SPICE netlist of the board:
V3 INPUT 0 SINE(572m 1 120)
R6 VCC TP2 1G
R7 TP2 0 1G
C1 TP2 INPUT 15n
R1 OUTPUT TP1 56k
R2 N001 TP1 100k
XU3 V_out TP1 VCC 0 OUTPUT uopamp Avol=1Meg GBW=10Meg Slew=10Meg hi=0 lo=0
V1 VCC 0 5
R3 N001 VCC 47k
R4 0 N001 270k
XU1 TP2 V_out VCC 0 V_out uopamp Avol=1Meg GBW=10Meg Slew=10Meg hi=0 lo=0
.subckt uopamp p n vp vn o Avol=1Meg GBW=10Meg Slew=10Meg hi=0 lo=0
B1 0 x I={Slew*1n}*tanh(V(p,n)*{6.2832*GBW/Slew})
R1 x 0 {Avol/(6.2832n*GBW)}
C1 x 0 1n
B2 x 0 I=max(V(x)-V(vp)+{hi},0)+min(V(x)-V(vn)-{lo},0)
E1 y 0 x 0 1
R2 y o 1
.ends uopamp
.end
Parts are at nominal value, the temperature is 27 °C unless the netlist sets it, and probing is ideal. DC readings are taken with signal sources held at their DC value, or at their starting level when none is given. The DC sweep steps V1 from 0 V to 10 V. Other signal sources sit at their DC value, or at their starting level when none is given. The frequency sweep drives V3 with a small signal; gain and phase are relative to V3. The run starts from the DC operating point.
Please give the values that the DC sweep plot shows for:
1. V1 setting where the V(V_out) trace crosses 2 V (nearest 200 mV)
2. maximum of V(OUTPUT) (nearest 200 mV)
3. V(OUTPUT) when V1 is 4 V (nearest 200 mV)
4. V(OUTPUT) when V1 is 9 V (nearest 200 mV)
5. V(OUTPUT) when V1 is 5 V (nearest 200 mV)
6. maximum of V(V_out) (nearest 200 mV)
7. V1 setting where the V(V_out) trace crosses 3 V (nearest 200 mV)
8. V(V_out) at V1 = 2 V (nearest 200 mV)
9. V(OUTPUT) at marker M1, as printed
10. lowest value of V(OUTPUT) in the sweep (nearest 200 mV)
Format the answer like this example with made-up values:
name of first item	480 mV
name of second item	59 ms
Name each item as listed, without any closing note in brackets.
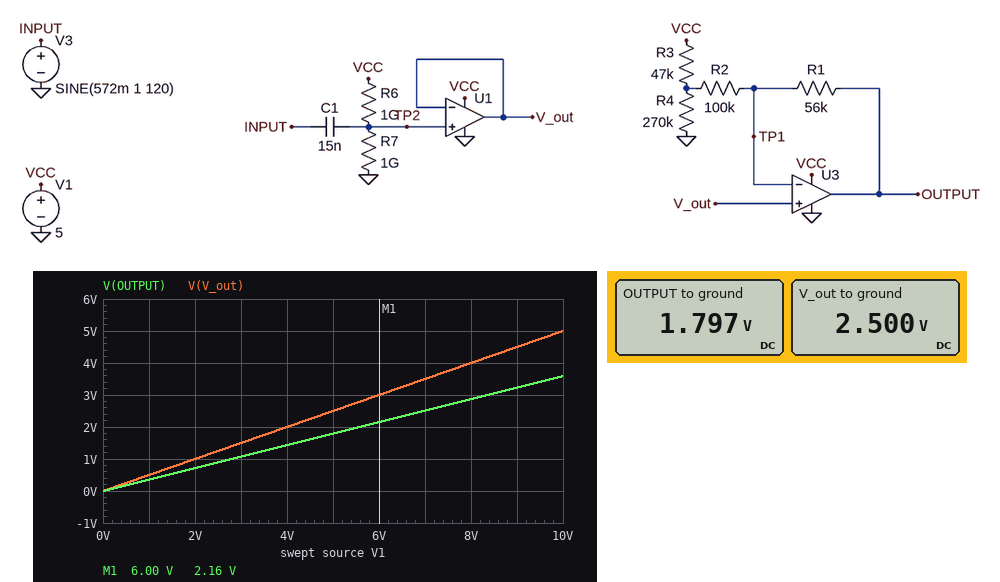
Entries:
V1 setting where the V(V_out) trace crosses 2 V	4.0 V
maximum of V(OUTPUT)	3.6 V
V(OUTPUT) when V1 is 4 V	1.4 V
V(OUTPUT) when V1 is 9 V	3.2 V
V(OUTPUT) when V1 is 5 V	1.8 V
maximum of V(V_out)	5.0 V
V1 setting where the V(V_out) trace crosses 3 V	6.0 V
V(V_out) at V1 = 2 V	1.0 V
V(OUTPUT) at marker M1, as printed	2.16 V
lowest value of V(OUTPUT) in the sweep	0 V
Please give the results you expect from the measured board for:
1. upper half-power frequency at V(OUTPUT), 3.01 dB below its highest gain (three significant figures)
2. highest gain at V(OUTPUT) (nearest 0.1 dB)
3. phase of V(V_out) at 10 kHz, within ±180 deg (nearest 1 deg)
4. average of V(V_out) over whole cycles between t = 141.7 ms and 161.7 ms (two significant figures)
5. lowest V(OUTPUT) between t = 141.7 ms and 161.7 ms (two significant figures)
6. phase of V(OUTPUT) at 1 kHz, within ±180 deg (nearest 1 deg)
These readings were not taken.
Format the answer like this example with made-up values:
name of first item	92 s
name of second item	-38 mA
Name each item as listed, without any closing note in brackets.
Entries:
upper half-power frequency at V(OUTPUT), 3.01 dB below its highest gain	5.33 MHz
highest gain at V(OUTPUT)	2.9 dB
phase of V(V_out) at 10 kHz, within ±180 deg	0 deg
average of V(V_out) over whole cycles between t = 141.7 ms and 161.7 ms	2.5 V
lowest V(OUTPUT) between t = 141.7 ms and 161.7 ms	400 mV
phase of V(OUTPUT) at 1 kHz, within ±180 deg	0 deg
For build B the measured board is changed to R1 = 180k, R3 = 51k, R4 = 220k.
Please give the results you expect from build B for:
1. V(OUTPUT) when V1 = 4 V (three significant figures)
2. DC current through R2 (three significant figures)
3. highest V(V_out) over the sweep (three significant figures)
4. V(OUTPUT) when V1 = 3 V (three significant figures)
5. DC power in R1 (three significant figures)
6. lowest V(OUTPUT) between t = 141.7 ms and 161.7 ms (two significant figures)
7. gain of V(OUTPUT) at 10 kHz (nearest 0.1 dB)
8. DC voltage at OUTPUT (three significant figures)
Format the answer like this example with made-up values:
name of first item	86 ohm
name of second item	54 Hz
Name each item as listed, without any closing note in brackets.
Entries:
V(OUTPUT) when V1 = 4 V	412 mV
DC current through R2	11.0 µA
highest V(V_out) over the sweep	5.00 V
V(OUTPUT) when V1 = 3 V	309 mV
DC power in R1	21.9 µW
lowest V(OUTPUT) between t = 141.7 ms and 161.7 ms	-10 mV
gain of V(OUTPUT) at 10 kHz	7.1 dB
DC voltage at OUTPUT	515 mV
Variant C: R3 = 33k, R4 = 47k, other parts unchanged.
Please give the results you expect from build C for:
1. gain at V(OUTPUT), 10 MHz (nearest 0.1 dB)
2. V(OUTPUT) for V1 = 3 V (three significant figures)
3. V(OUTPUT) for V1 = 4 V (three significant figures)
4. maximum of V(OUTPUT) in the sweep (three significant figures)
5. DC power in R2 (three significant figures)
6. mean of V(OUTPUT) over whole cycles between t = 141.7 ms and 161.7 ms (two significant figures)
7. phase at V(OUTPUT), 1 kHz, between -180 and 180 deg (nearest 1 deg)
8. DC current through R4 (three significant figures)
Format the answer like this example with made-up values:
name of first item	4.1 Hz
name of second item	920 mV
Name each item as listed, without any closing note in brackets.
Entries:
gain at V(OUTPUT), 10 MHz	-4.7 dB
V(OUTPUT) for V1 = 3 V	1.38 V
V(OUTPUT) for V1 = 4 V	1.84 V
maximum of V(OUTPUT) in the sweep	4.59 V
DC power in R2	1.34 µW
mean of V(OUTPUT) over whole cycles between t = 141.7 ms and 161.7 ms	2.3 V
phase at V(OUTPUT), 1 kHz, between -180 and 180 deg	0 deg
DC current through R4	61.0 µA
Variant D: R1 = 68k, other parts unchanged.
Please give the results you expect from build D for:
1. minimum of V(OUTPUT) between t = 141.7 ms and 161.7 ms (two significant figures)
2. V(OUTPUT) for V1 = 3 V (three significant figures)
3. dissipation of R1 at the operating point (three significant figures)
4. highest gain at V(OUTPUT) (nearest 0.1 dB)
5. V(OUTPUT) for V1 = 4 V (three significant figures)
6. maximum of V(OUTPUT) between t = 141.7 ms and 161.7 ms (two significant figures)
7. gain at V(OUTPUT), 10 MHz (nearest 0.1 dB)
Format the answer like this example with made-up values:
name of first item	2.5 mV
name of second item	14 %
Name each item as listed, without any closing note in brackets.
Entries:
minimum of V(OUTPUT) between t = 141.7 ms and 161.7 ms	160 mV
V(OUTPUT) for V1 = 3 V	988 mV
dissipation of R1 at the operating point	10.7 µW
highest gain at V(OUTPUT)	3.4 dB
V(OUTPUT) for V1 = 4 V	1.32 V
maximum of V(OUTPUT) between t = 141.7 ms and 161.7 ms	3.1 V
gain at V(OUTPUT), 10 MHz	-4.6 dB
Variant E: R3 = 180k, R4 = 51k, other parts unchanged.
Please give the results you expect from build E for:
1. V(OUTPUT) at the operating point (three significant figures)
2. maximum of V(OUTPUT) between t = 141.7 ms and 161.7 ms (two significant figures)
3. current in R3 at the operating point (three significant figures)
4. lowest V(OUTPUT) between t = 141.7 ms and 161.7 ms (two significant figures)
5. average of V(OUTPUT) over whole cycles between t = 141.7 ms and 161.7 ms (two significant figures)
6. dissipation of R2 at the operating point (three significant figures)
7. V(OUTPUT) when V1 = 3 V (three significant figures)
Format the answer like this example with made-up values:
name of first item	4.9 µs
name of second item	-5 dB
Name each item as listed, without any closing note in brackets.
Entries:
V(OUTPUT) at the operating point	3.06 V
maximum of V(OUTPUT) between t = 141.7 ms and 161.7 ms	4.5 V
current in R3 at the operating point	19.4 µA
lowest V(OUTPUT) between t = 141.7 ms and 161.7 ms	1.7 V
average of V(OUTPUT) over whole cycles between t = 141.7 ms and 161.7 ms	3.1 V
dissipation of R2 at the operating point	9.98 µW
V(OUTPUT) when V1 = 3 V	1.84 V
